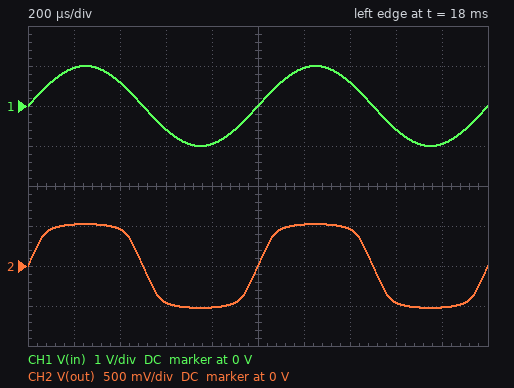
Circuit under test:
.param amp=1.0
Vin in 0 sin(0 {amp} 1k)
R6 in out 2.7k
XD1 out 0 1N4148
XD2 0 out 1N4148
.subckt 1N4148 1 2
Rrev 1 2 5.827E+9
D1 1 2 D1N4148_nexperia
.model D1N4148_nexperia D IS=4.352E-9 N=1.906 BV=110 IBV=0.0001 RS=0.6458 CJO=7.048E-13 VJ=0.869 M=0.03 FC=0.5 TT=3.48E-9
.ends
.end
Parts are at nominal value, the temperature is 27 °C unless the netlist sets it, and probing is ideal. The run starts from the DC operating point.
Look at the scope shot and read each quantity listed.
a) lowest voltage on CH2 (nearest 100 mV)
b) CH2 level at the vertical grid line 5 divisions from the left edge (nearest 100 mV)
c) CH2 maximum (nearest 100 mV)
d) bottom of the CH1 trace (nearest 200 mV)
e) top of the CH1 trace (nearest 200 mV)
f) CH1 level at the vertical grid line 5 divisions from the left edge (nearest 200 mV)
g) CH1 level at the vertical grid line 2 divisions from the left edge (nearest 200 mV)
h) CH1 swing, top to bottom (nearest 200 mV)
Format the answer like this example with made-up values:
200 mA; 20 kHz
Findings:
-500 mV; 0 V; 500 mV; -1.0 V; 1.0 V; 0 V; 600 mV; 2.0 V
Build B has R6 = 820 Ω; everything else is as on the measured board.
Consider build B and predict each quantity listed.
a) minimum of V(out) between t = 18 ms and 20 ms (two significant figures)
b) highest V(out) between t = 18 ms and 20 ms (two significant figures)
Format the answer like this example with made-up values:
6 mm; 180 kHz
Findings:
-580 mV; 580 mV
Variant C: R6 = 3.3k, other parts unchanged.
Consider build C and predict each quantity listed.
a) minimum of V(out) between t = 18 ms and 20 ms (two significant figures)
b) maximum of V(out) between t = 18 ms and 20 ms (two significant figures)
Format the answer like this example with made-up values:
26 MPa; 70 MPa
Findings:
-510 mV; 510 mV
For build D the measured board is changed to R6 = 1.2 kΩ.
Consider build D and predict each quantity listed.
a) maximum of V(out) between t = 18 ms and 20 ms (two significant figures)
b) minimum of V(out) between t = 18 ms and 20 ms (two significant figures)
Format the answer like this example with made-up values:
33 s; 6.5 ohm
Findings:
560 mV; -560 mV
